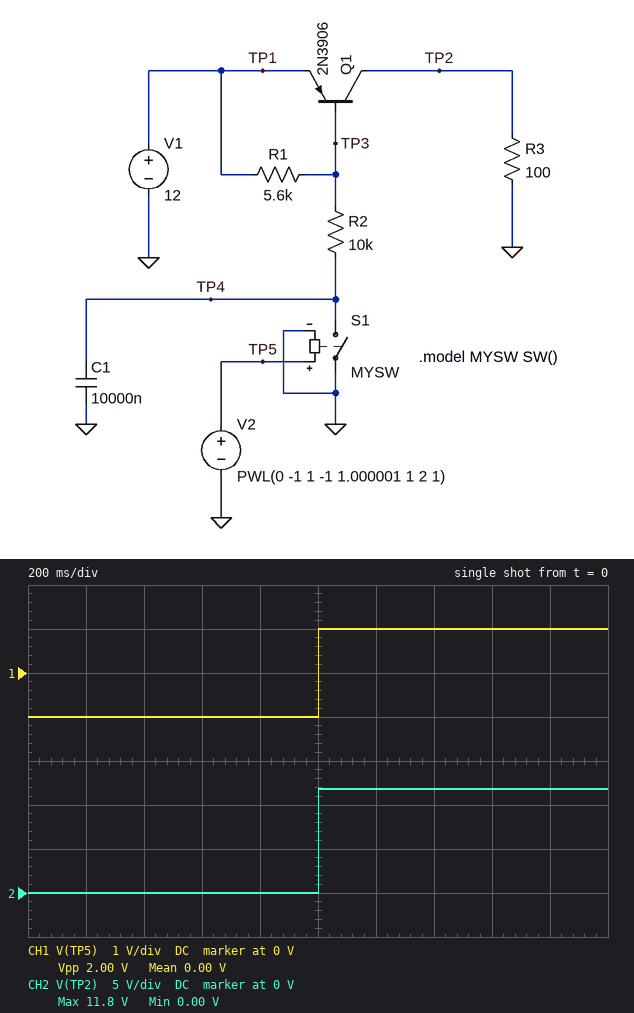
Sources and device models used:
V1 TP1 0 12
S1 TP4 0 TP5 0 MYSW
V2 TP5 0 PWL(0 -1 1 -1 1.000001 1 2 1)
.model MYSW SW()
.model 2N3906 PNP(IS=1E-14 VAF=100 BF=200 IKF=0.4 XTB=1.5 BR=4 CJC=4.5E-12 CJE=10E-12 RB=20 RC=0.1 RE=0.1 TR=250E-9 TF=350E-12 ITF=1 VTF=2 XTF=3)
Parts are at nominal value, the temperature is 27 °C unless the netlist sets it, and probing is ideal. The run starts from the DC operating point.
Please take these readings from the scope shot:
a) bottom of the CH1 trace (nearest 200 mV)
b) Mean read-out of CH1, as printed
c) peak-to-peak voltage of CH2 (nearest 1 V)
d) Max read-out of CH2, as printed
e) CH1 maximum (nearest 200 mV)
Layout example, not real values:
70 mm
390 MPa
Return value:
-1.0 V
0.00 V
12 V
11.8 V
1.0 V
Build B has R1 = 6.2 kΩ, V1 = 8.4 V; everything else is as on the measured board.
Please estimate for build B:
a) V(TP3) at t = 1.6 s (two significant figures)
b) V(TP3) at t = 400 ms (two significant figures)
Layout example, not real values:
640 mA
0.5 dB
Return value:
7.6 V
8.4 V
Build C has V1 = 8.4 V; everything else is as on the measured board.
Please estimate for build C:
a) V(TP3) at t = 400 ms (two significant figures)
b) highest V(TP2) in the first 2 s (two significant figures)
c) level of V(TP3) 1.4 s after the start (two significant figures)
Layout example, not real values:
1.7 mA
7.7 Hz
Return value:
8.4 V
8.2 V
7.6 V
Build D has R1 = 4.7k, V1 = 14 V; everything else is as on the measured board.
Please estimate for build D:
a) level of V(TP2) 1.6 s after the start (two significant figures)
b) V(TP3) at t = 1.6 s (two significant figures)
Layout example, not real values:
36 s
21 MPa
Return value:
14 V
13 V
